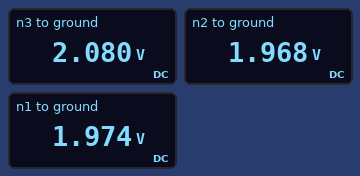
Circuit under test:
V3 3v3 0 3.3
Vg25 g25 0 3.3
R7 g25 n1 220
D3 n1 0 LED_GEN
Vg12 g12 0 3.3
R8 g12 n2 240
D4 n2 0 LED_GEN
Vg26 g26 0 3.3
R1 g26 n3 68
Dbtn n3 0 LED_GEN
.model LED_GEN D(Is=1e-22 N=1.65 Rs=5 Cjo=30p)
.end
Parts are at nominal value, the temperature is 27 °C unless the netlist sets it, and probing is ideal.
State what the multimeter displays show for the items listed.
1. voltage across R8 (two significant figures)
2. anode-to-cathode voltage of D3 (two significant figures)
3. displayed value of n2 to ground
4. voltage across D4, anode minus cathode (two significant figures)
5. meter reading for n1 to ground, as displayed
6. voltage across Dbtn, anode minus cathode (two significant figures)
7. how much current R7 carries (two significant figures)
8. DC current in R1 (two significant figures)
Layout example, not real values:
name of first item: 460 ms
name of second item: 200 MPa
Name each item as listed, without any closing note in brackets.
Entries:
voltage across R8: 1.3 V
anode-to-cathode voltage of D3: 2.0 V
displayed value of n2 to ground: 1.968 V
voltage across D4, anode minus cathode: 2.0 V
meter reading for n1 to ground, as displayed: 1.974 V
voltage across Dbtn, anode minus cathode: 2.1 V
how much current R7 carries: 6.0 mA
DC current in R1: 18 mA
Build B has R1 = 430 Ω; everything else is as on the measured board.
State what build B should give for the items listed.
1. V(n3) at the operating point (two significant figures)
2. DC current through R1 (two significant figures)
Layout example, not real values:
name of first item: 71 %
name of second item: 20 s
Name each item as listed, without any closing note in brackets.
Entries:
V(n3) at the operating point: 1.9 V
DC current through R1: 3.2 mA
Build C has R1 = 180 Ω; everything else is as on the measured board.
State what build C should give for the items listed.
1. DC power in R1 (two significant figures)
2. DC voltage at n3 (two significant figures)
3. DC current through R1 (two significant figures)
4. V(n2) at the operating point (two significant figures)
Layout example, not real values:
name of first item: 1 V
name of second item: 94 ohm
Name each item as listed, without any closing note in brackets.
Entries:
DC power in R1: 9.6 mW
DC voltage at n3: 2.0 V
DC current through R1: 7.3 mA
V(n2) at the operating point: 2.0 V
